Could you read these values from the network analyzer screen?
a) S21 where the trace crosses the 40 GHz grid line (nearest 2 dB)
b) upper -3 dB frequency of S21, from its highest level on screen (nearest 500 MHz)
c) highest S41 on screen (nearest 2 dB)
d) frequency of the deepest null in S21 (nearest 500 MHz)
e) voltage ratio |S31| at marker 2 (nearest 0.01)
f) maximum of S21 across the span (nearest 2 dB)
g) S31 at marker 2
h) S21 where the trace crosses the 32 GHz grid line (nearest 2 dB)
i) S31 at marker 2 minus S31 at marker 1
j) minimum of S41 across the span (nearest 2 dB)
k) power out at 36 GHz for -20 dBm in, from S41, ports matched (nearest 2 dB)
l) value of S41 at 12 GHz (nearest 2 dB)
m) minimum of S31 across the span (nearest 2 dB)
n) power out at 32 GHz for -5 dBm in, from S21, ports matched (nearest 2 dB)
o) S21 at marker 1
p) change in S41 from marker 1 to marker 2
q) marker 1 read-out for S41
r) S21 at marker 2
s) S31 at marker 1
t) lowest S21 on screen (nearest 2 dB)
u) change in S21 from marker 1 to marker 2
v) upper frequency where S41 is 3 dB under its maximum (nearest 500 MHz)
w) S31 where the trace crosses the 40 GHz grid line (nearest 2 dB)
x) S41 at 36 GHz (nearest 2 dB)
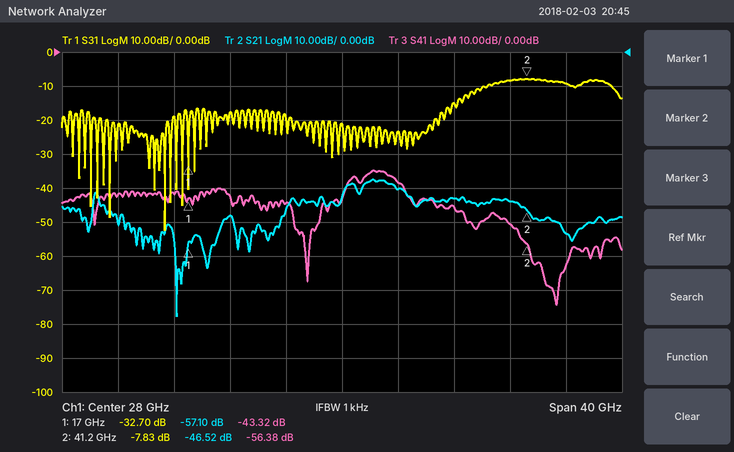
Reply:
-44 dB
32.5 GHz
-34 dB
16.0 GHz
0.41
-38 dB
-7.83 dB
-40 dB
24.87 dB
-74 dB
-66 dBm
-42 dB
-52 dB
-46 dBm
-57.10 dB
-13.06 dB
-43.32 dB
-46.52 dB
-32.70 dB
-78 dB
10.58 dB
32.0 GHz
-8 dB
-46 dB
